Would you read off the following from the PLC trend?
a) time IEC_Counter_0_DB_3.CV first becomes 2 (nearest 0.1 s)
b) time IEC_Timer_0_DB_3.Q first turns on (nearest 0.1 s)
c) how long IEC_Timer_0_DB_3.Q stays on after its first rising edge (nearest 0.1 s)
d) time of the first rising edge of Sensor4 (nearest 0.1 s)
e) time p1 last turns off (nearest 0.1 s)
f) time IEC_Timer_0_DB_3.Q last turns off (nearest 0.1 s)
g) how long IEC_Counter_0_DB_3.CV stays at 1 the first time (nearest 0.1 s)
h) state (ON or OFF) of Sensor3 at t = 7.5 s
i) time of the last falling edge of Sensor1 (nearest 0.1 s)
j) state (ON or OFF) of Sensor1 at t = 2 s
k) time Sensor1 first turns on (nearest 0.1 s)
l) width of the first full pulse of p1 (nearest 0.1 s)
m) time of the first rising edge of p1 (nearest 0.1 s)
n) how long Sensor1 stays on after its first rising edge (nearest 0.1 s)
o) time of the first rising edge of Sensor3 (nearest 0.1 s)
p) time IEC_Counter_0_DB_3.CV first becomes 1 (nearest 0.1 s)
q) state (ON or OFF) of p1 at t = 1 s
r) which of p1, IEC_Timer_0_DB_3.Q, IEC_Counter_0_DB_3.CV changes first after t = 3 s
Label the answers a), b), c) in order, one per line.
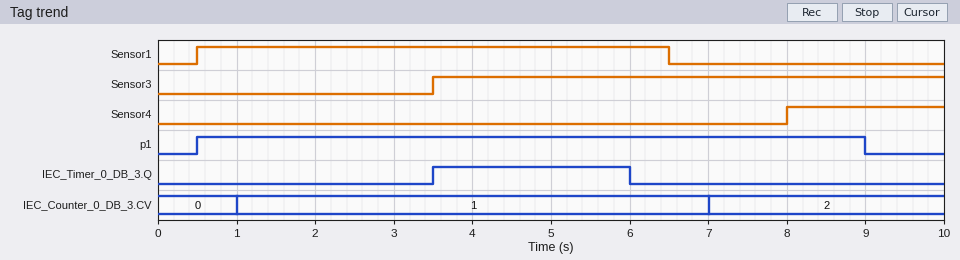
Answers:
a) 7.0 s
b) 3.5 s
c) 2.5 s
d) 8.0 s
e) 9.0 s
f) 6.0 s
g) 6.0 s
h) ON
i) 6.5 s
j) ON
k) 0.5 s
l) 8.5 s
m) 0.5 s
n) 6.0 s
o) 3.5 s
p) 1.0 s
q) ON
r) IEC_Timer_0_DB_3.Q
